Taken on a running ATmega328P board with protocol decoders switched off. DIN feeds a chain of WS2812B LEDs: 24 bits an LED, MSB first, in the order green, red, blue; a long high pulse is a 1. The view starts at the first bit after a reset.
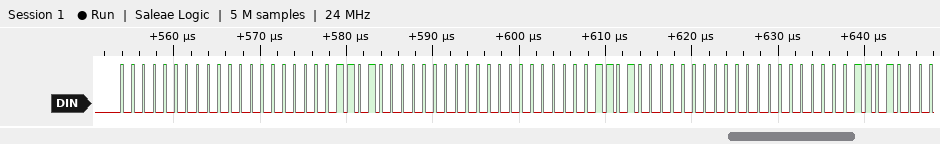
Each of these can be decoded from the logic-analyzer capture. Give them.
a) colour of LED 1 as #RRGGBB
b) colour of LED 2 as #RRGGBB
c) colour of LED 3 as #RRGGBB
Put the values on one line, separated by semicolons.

#00000D; #00000D; #00000D
